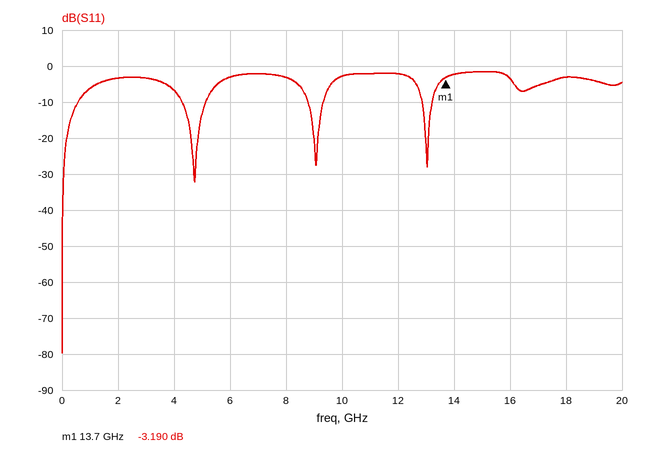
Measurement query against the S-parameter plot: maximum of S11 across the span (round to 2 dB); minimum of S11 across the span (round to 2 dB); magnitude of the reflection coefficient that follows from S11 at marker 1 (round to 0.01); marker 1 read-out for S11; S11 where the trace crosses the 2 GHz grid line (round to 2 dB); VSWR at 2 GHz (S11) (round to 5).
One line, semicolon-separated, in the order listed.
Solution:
-2 dB; -80 dB; 0.69; -3.190 dB; -4 dB; 5
